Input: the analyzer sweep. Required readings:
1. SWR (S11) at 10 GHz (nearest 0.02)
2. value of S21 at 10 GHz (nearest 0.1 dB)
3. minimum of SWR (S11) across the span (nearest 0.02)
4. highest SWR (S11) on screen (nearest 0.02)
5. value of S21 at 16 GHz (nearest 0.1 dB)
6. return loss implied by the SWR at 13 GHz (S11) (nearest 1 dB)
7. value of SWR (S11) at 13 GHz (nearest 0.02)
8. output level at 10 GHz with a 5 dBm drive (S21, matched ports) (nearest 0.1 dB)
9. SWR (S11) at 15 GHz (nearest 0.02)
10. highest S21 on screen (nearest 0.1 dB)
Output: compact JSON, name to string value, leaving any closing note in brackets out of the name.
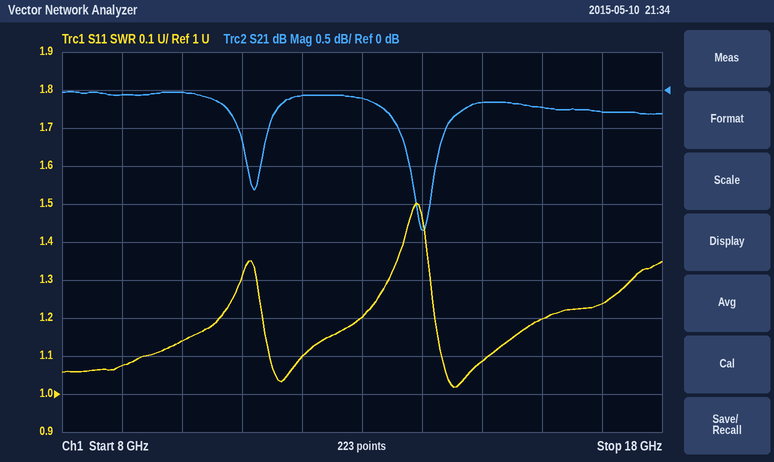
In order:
{"SWR (S11) at 10 GHz": "1.14", "value of S21 at 10 GHz": "0.0 dB", "minimum of SWR (S11) across the span": "1.02", "highest SWR (S11) on screen": "1.50", "value of S21 at 16 GHz": "-0.2 dB", "return loss implied by the SWR at 13 GHz (S11)": "21 dB", "value of SWR (S11) at 13 GHz": "1.20", "output level at 10 GHz with a 5 dBm drive (S21, matched ports)": "5.0 dBm", "SWR (S11) at 15 GHz": "1.08", "highest S21 on screen": "0.0 dB"}
